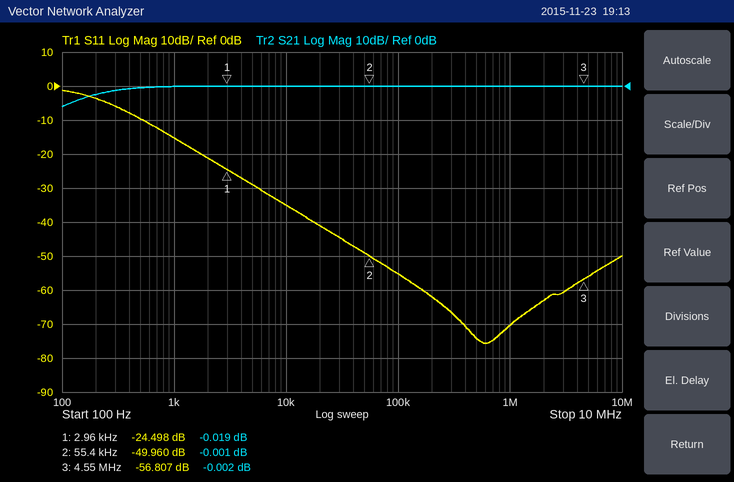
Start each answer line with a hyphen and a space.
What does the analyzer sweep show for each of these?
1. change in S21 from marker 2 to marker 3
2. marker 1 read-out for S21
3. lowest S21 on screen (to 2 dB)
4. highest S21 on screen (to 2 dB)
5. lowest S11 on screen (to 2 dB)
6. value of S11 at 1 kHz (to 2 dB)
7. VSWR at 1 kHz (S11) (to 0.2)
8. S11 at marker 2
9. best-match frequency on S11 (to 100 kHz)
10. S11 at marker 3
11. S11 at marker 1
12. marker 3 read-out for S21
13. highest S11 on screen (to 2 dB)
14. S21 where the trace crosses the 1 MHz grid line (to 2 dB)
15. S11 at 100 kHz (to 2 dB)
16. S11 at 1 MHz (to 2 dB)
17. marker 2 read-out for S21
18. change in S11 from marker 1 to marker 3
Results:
- -0.001 dB
- -0.019 dB
- -6 dB
- 0 dB
- -76 dB
- -16 dB
- 1.4
- -49.960 dB
- 600 kHz
- -56.807 dB
- -24.498 dB
- -0.002 dB
- -2 dB
- 0 dB
- -56 dB
- -70 dB
- -0.001 dB
- -32.309 dB
